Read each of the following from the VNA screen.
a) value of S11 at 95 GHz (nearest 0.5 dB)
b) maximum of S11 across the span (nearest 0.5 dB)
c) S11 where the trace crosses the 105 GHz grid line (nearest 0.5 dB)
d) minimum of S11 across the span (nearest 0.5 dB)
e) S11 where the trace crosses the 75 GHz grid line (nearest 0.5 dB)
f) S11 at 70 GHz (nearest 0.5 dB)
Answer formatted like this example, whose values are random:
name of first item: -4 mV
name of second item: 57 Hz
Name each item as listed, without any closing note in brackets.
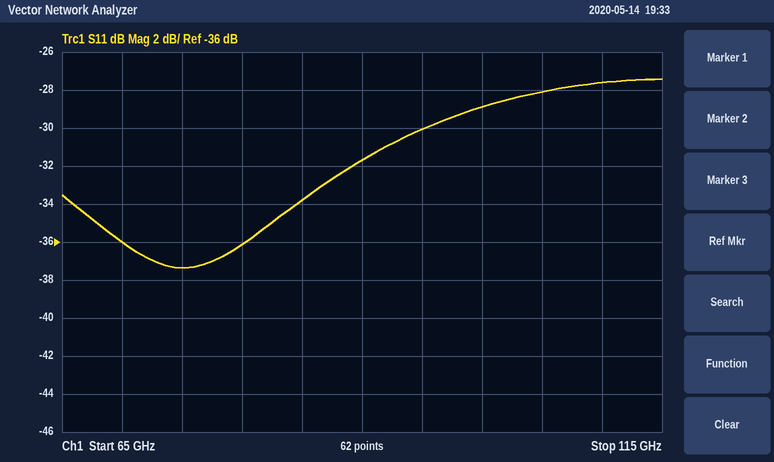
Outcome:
value of S11 at 95 GHz: -30.0 dB
maximum of S11 across the span: -27.5 dB
S11 where the trace crosses the 105 GHz grid line: -28.0 dB
minimum of S11 across the span: -37.5 dB
S11 where the trace crosses the 75 GHz grid line: -37.5 dB
S11 at 70 GHz: -36.0 dB
